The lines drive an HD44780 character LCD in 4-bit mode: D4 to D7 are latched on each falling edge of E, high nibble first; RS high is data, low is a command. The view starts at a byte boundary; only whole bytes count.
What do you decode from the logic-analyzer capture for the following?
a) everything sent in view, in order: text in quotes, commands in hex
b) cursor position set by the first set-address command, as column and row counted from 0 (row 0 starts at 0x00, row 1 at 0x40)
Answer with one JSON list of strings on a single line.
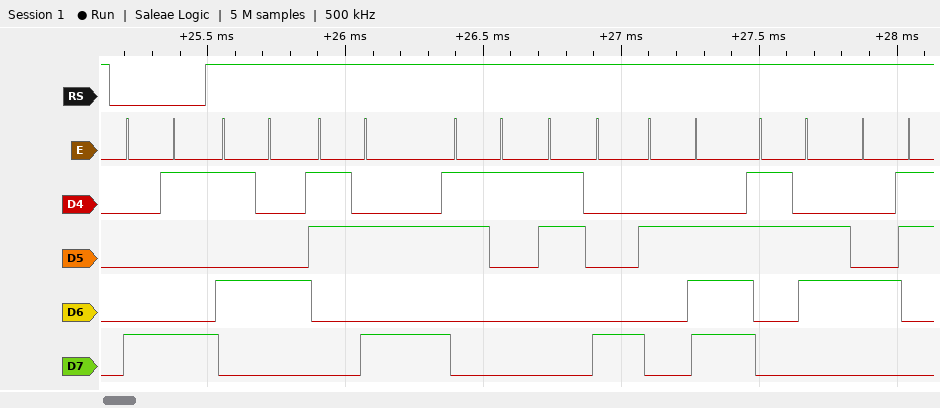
["0x89 \"T:18.6C\"", "column 9, row 0"]
